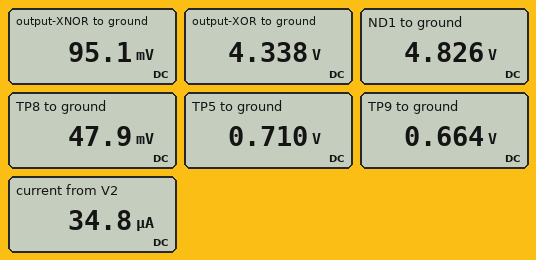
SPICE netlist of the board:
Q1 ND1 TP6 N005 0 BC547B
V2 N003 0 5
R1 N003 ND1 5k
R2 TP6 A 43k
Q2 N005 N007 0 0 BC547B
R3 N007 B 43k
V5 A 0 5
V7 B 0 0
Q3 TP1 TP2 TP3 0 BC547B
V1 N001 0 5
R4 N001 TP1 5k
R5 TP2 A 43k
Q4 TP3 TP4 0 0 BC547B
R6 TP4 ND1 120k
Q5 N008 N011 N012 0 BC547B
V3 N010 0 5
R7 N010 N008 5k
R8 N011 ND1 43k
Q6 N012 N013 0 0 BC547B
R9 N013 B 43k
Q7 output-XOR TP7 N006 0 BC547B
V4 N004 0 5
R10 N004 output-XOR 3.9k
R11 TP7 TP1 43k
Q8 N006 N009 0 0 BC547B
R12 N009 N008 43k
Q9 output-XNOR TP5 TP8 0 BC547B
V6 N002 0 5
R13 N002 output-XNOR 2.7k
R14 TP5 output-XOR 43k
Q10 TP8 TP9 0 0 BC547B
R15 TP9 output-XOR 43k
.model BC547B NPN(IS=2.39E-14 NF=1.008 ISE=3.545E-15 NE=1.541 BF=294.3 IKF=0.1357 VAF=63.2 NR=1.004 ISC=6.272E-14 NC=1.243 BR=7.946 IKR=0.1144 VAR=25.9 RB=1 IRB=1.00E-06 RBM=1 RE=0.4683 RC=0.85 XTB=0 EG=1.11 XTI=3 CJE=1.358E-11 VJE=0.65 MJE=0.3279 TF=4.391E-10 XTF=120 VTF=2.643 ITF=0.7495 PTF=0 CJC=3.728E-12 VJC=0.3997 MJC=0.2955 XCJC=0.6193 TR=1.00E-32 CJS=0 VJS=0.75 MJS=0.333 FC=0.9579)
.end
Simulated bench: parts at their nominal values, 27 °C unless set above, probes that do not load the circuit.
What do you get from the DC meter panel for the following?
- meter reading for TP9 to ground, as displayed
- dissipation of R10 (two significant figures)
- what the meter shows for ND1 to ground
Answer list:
0.664 V
110 µW
4.826 V
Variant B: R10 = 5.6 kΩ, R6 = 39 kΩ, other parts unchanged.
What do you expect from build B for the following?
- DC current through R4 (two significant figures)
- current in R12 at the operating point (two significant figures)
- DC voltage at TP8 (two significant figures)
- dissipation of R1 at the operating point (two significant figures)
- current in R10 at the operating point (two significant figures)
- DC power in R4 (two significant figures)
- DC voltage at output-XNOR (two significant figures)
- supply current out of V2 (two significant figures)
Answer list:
990 µA
91 µA
49 mV
48 µW
160 µA
4.9 mW
98 mV
98 µA
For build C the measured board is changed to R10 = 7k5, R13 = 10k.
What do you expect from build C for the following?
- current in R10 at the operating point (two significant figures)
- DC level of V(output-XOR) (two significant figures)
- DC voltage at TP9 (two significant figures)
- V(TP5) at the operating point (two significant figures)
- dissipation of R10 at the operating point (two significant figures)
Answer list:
150 µA
3.9 V
640 mV
670 mV
170 µW
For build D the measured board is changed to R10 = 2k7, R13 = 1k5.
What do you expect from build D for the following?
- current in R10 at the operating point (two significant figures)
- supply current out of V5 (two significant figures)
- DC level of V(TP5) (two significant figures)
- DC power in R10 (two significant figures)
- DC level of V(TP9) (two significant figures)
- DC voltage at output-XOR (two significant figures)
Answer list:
180 µA
100 µA
740 mV
85 µW
680 mV
4.5 V
